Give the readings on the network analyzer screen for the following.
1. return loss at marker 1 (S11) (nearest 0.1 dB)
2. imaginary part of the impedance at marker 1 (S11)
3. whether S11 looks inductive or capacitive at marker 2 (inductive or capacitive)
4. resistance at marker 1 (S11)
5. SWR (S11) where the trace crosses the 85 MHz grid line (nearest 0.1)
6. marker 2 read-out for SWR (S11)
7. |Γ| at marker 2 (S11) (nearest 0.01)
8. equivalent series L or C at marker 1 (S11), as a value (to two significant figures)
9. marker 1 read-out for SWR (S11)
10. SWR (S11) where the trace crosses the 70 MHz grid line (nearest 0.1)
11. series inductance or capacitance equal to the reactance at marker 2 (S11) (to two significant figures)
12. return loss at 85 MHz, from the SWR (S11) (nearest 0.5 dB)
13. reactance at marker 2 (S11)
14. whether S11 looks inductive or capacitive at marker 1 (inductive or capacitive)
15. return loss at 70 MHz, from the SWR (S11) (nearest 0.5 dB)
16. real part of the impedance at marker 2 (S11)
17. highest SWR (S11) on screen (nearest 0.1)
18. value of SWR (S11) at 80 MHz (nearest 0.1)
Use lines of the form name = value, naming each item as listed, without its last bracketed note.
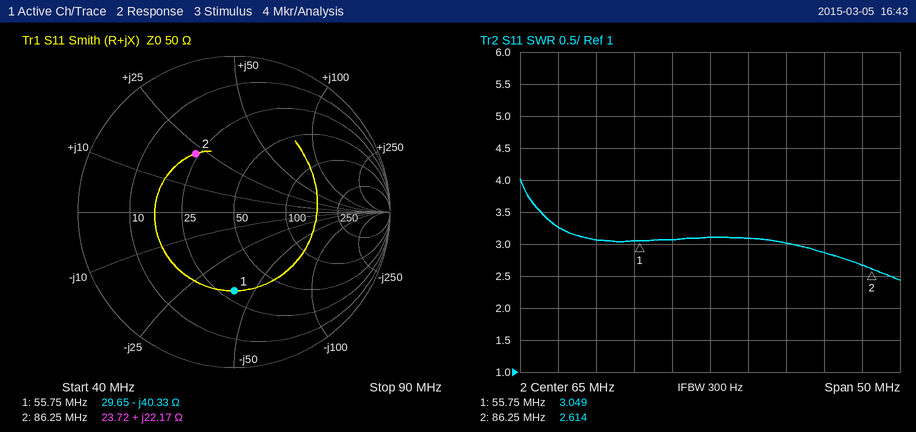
return loss at marker 1 (S11) = 5.9 dB
imaginary part of the impedance at marker 1 = -40.33 Ω
whether S11 looks inductive or capacitive at marker 2 = inductive
resistance at marker 1 = 29.65 Ω
SWR (S11) where the trace crosses the 85 MHz grid line = 2.7
marker 2 read-out for SWR = 2.614
|Γ| at marker 2 (S11) = 0.45
equivalent series L or C at marker 1 (S11), as a value = 71 pF
marker 1 read-out for SWR = 3.049
SWR (S11) where the trace crosses the 70 MHz grid line = 3.1
series inductance or capacitance equal to the reactance at marker 2 (S11) = 41 nH
return loss at 85 MHz, from the SWR (S11) = 7.0 dB
reactance at marker 2 = +22.17 Ω
whether S11 looks inductive or capacitive at marker 1 = capacitive
return loss at 70 MHz, from the SWR (S11) = 6.0 dB
real part of the impedance at marker 2 = 23.72 Ω
highest SWR (S11) on screen = 4.0
value of SWR (S11) at 80 MHz = 2.9
